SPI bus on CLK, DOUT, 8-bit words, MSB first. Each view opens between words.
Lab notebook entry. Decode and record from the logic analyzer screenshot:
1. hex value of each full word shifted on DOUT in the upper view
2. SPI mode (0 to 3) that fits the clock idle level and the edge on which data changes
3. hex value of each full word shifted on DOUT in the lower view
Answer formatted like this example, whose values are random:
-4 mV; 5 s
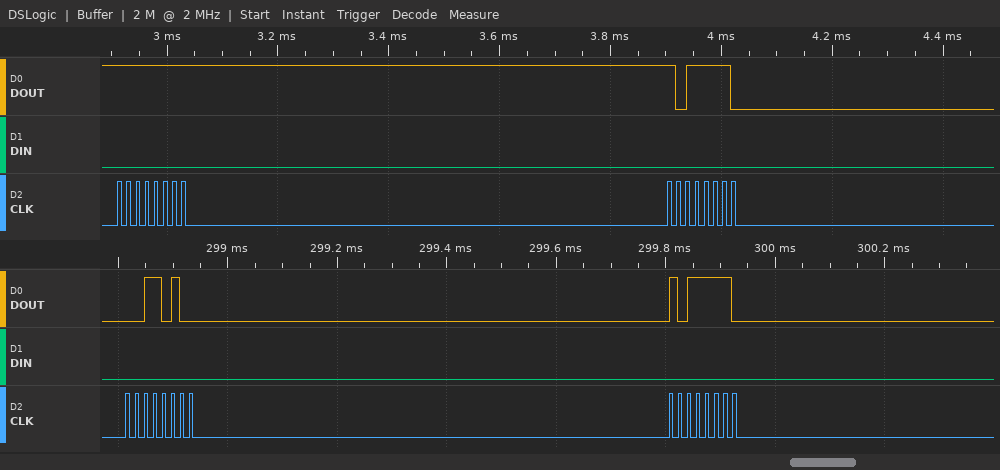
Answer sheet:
FF, BE; 1; 34, BE
